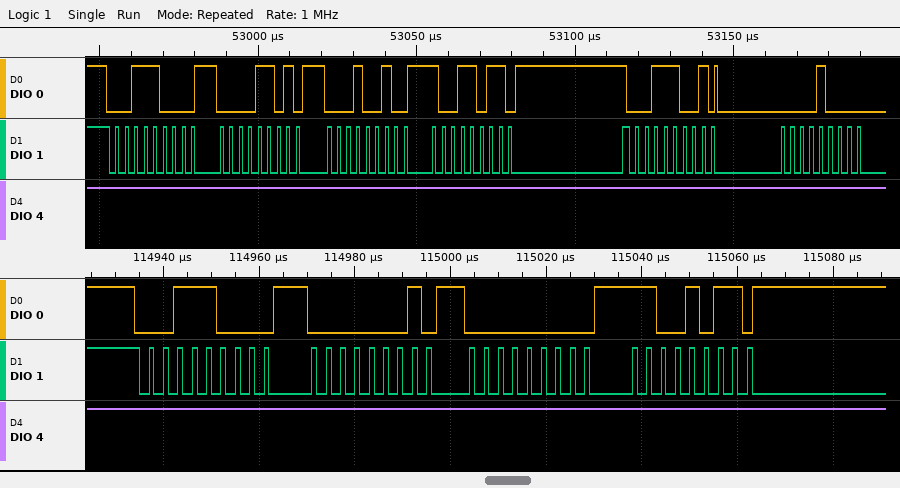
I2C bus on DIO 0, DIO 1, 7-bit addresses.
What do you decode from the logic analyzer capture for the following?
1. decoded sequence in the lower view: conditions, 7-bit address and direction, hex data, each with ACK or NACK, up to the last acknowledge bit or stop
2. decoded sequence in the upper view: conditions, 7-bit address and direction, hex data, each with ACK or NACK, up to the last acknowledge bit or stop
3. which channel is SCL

start, address 1C write ACK, 01 ACK, 00 ACK, CB ACK
start, address 1C write ACK, 0D ACK, 12 ACK, 9B ACK, repeated start, address 1C read ACK, 08 ACK
DIO 1
